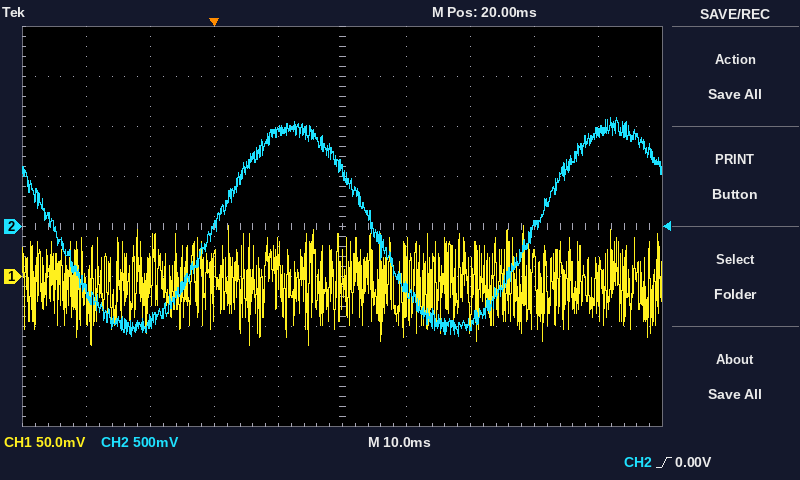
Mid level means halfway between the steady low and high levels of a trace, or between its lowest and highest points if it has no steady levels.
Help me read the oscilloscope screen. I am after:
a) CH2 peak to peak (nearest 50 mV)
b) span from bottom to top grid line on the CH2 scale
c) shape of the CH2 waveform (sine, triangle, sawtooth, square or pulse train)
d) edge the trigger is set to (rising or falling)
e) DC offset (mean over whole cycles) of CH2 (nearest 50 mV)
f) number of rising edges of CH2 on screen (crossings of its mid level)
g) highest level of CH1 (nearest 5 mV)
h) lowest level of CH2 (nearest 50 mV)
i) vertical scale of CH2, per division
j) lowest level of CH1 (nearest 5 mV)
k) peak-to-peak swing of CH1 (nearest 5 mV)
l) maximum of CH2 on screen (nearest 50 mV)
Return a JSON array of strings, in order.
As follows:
["2.20 V", "4 V", "sine", "rising", "0 mV", "2", "50 mV", "-1.10 V", "500 mV", "-70 mV", "120 mV", "1.10 V"]
